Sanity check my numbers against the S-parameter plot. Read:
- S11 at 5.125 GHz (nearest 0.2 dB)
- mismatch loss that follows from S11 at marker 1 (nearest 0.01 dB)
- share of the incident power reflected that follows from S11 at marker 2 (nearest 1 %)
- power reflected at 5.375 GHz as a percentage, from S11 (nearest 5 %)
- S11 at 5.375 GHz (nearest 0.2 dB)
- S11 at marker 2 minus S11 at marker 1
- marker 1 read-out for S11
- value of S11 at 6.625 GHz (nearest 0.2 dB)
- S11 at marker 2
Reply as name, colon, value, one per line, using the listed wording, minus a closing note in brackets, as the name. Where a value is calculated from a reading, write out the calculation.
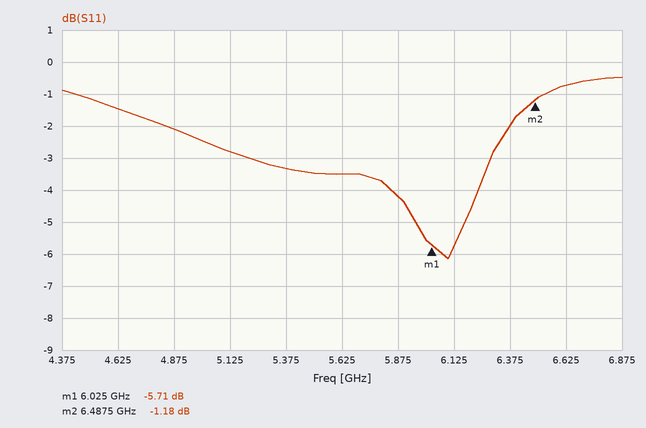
S11 at 5.125 GHz: -2.8 dB
mismatch loss that follows from S11 at marker 1: −10 log10(1 − 10^(-5.71/10)) ≈ 1.36 dB
share of the incident power reflected that follows from S11 at marker 2: 10^(-1.18/10) ≈ 76 %
power reflected at 5.375 GHz as a percentage, from S11: 10^(-3.4/10) ≈ 45.7 %, so 45 % to the nearest 5 %
S11 at 5.375 GHz: -3.4 dB
S11 at marker 2 minus S11 at marker 1: -1.18 − (-5.71) = 4.53 dB
marker 1 read-out for S11: -5.71 dB
value of S11 at 6.625 GHz: -0.8 dB
S11 at marker 2: -1.18 dB
